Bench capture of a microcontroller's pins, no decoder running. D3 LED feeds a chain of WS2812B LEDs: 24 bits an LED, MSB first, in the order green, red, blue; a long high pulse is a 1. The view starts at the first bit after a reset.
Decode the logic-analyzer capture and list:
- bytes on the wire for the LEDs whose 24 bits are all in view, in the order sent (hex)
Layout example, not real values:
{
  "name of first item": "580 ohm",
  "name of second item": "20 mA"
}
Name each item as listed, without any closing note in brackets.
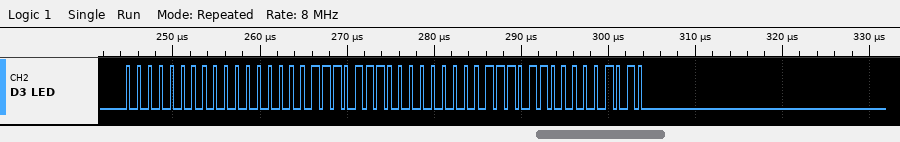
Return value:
{
  "bytes on the wire for the LEDs whose 24 bits are all in view, in the order sent": "00 00 77 00 76 0A"
}
